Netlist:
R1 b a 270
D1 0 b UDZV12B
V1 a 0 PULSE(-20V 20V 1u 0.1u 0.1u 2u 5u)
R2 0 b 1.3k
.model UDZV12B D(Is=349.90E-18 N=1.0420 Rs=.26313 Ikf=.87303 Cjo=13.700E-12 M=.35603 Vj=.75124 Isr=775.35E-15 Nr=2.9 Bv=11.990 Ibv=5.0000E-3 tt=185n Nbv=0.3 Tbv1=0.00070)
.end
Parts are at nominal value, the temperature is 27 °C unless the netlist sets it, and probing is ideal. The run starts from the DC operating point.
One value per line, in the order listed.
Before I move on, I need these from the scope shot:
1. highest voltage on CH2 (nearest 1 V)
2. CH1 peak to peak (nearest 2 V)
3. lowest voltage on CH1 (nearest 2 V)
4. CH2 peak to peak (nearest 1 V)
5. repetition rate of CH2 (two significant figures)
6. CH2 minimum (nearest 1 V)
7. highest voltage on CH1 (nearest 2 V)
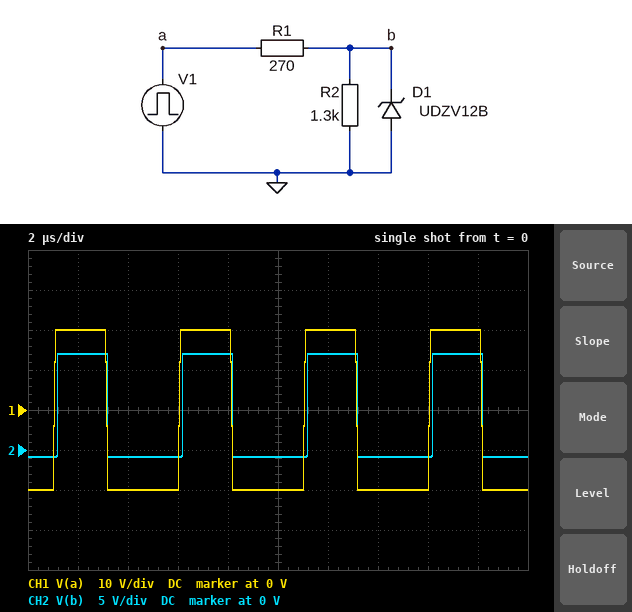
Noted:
12 V
40 V
-20 V
13 V
200 kHz
-1 V
20 V
